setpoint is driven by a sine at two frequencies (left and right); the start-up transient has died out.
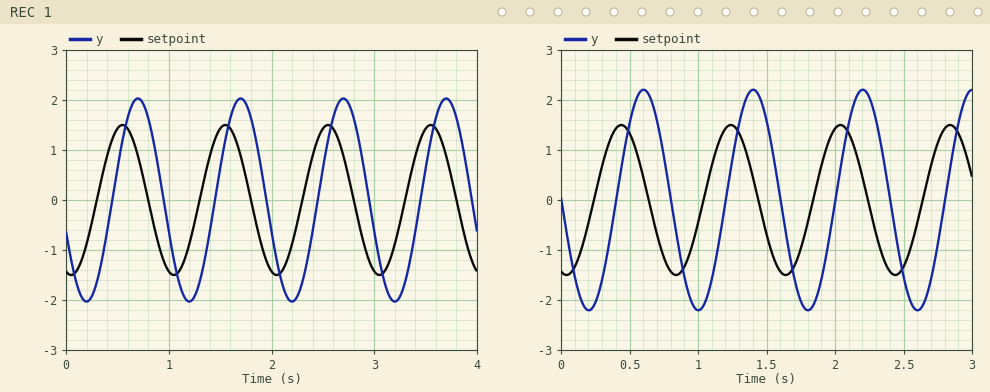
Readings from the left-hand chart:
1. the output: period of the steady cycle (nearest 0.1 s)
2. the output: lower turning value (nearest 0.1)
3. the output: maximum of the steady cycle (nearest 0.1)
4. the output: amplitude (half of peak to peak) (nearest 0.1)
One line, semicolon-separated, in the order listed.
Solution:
1.0 s; -2.0; 2.0; 2.0
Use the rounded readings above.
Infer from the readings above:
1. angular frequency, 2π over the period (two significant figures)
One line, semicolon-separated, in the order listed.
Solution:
6.3 rad/s
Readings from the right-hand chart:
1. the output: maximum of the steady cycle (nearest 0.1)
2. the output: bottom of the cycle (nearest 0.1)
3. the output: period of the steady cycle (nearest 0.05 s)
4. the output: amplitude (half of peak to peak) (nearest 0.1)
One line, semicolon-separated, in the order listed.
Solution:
2.2; -2.2; 0.80 s; 2.2
